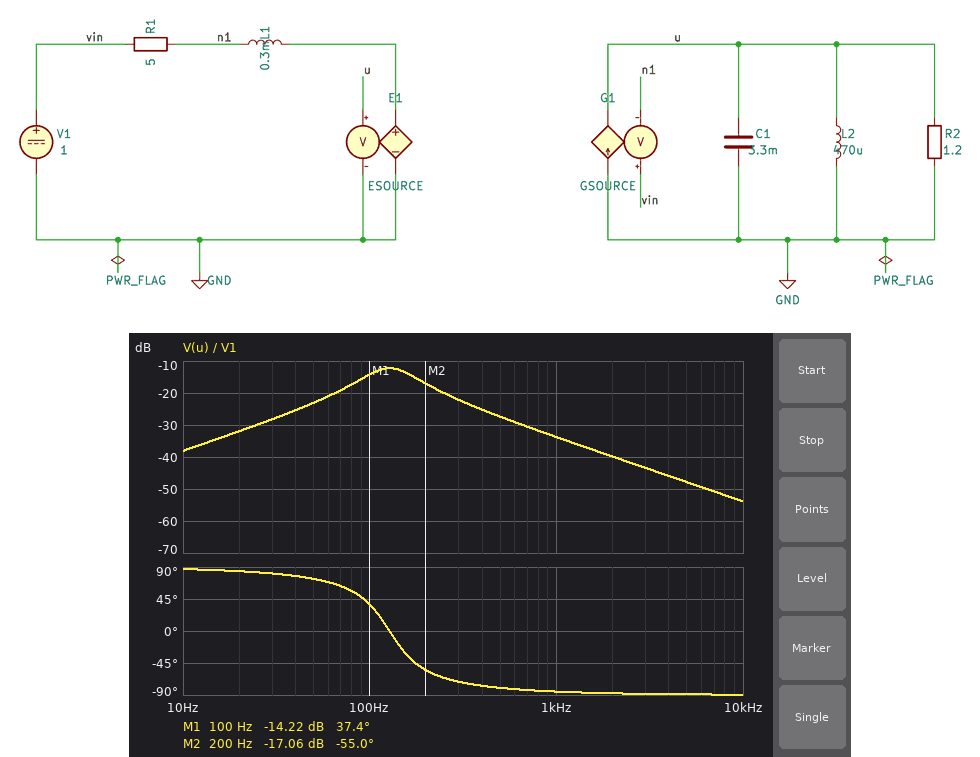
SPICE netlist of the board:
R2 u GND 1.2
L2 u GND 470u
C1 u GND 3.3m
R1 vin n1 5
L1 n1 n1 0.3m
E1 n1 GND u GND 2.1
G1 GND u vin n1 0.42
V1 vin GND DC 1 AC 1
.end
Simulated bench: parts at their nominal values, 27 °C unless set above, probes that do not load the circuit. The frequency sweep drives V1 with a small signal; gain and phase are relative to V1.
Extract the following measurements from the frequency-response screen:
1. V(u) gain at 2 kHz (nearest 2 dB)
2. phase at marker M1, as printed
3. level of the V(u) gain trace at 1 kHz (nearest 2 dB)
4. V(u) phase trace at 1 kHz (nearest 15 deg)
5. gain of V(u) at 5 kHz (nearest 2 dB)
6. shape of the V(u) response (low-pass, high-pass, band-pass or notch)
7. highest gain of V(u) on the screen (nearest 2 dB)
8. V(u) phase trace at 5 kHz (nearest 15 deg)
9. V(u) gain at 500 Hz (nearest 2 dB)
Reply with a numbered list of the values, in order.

1. -40 dB
2. 37.4 deg
3. -34 dB
4. -90 deg
5. -48 dB
6. band-pass
7. -12 dB
8. -90 deg
9. -28 dB
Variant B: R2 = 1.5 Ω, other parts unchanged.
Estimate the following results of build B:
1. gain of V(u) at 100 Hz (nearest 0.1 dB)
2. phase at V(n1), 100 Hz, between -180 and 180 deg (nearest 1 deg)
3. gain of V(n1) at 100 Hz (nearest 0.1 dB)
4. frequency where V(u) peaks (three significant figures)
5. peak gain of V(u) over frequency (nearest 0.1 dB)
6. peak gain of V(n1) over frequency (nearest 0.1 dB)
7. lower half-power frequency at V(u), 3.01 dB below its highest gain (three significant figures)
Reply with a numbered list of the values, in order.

1. -13.7 dB
2. 40 deg
3. -7.2 dB
4. 128 Hz
5. -11.3 dB
6. -4.9 dB
7. 95.8 Hz
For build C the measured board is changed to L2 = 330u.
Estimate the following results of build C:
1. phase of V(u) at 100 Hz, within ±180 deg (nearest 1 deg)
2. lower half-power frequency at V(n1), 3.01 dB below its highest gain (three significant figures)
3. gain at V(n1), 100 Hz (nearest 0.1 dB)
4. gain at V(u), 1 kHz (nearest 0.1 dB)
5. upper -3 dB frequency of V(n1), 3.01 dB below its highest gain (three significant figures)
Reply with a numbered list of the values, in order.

1. 58 deg
2. 117 Hz
3. -11.3 dB
4. -33.7 dB
5. 199 Hz
